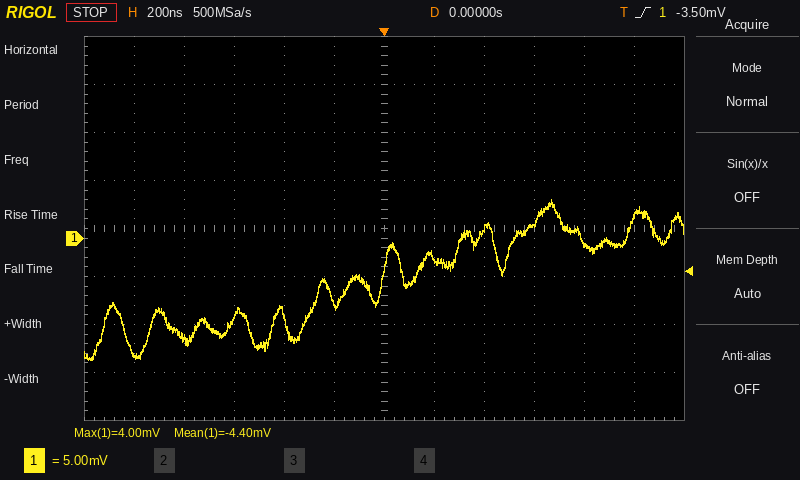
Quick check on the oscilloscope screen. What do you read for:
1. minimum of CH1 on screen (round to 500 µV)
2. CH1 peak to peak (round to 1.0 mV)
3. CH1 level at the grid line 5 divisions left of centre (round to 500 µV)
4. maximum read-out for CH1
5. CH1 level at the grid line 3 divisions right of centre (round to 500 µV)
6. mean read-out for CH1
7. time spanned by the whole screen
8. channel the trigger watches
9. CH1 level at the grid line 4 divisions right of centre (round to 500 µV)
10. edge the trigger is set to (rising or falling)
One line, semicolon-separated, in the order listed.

-12.5 mV; 17.0 mV; -12.0 mV; 4.00 mV; 1.5 mV; -4.40 mV; 2.4 µs; CH1; -500 µV; rising
